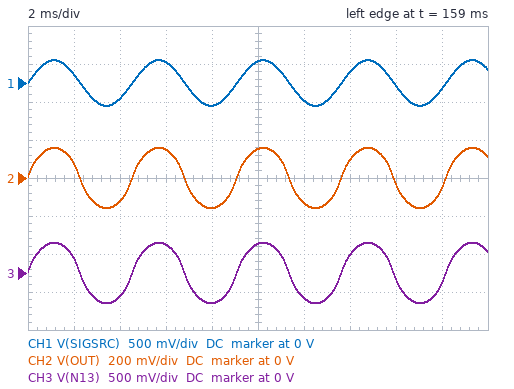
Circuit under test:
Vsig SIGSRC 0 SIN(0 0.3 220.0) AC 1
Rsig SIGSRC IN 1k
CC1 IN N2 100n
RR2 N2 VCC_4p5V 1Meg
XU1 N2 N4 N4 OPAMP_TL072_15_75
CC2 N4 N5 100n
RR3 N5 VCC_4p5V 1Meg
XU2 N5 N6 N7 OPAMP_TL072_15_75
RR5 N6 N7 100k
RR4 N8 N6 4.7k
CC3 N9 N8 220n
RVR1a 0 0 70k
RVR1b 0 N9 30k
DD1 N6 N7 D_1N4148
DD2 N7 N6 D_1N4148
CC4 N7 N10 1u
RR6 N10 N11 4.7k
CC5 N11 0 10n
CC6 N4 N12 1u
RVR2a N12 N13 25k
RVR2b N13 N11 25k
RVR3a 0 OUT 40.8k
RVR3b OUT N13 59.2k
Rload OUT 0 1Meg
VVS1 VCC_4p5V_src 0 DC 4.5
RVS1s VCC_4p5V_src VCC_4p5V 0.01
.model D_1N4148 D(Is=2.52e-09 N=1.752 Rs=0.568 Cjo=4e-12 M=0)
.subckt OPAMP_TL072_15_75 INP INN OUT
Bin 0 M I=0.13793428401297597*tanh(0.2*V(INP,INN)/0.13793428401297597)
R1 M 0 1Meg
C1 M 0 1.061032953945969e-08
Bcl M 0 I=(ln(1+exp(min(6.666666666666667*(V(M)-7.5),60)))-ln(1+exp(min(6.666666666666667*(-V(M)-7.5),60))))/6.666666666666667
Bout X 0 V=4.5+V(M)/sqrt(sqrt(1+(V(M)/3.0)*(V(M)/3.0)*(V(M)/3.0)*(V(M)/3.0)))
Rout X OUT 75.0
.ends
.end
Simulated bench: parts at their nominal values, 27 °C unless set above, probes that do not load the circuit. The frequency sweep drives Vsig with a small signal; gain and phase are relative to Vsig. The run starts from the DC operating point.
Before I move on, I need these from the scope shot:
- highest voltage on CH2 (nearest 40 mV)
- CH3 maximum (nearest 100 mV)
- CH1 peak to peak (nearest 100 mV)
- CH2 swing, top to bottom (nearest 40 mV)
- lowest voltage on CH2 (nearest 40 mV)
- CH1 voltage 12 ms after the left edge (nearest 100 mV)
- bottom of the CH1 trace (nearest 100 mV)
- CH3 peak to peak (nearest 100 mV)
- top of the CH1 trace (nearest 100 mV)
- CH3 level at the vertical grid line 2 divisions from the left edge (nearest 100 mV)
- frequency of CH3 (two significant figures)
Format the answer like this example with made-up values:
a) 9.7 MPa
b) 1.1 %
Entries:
a) 160 mV
b) 400 mV
c) 600 mV
d) 320 mV
e) -160 mV
f) -200 mV
g) -300 mV
h) 800 mV
i) 300 mV
j) -300 mV
k) 220 Hz
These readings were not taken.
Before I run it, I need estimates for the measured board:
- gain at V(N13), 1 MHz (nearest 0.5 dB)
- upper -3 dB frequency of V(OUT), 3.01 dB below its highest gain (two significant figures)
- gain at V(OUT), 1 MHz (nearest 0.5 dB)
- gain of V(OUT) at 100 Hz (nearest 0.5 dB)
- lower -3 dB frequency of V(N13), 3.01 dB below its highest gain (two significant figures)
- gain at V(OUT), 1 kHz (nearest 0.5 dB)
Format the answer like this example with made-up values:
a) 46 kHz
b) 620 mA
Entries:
a) -7.5 dB
b) 4.0 kHz
c) -15.5 dB
d) -2.0 dB
e) 17 Hz
f) -2.0 dB
